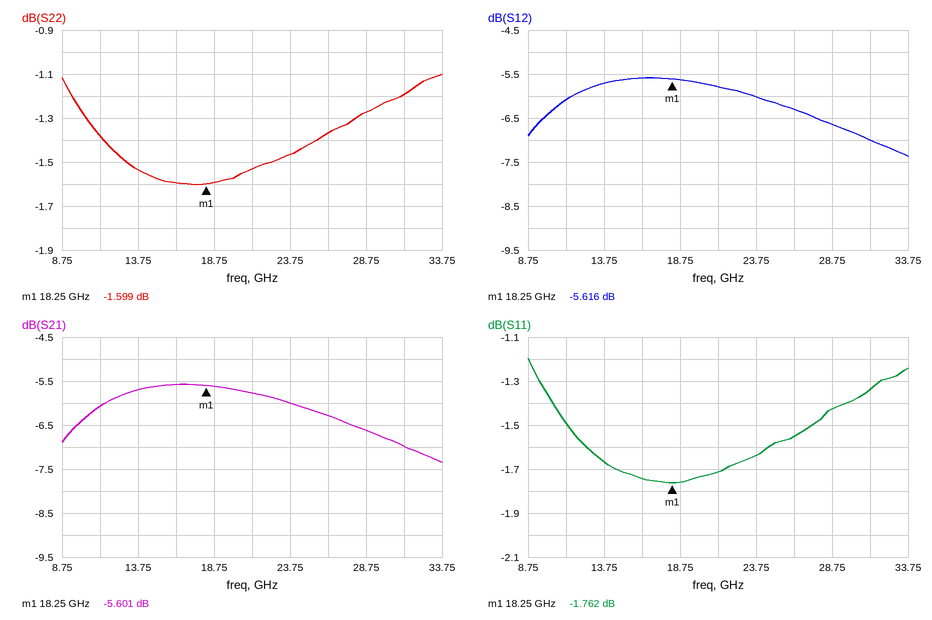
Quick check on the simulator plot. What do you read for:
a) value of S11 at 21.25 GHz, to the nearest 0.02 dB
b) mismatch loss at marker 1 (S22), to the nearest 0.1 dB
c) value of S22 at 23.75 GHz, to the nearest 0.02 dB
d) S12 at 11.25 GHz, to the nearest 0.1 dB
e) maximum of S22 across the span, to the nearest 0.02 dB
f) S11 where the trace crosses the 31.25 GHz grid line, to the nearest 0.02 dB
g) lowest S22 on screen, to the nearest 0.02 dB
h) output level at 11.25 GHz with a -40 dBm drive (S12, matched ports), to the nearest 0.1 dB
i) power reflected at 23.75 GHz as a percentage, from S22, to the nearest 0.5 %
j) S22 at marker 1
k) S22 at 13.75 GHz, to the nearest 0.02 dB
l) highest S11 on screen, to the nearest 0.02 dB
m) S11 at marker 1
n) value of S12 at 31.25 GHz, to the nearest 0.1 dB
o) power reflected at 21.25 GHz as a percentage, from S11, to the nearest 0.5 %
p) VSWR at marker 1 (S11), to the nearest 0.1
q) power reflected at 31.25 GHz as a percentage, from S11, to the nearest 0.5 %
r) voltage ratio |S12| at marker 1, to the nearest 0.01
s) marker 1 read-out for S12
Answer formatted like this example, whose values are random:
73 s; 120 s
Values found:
-1.72 dB; 5.1 dB; -1.46 dB; -6.1 dB; -1.10 dB; -1.34 dB; -1.60 dB; -46.1 dBm; 71.5 %; -1.599 dB; -1.54 dB; -1.20 dB; -1.762 dB; -7.0 dB; 67.5 %; 9.9; 73.5 %; 0.52; -5.616 dB
